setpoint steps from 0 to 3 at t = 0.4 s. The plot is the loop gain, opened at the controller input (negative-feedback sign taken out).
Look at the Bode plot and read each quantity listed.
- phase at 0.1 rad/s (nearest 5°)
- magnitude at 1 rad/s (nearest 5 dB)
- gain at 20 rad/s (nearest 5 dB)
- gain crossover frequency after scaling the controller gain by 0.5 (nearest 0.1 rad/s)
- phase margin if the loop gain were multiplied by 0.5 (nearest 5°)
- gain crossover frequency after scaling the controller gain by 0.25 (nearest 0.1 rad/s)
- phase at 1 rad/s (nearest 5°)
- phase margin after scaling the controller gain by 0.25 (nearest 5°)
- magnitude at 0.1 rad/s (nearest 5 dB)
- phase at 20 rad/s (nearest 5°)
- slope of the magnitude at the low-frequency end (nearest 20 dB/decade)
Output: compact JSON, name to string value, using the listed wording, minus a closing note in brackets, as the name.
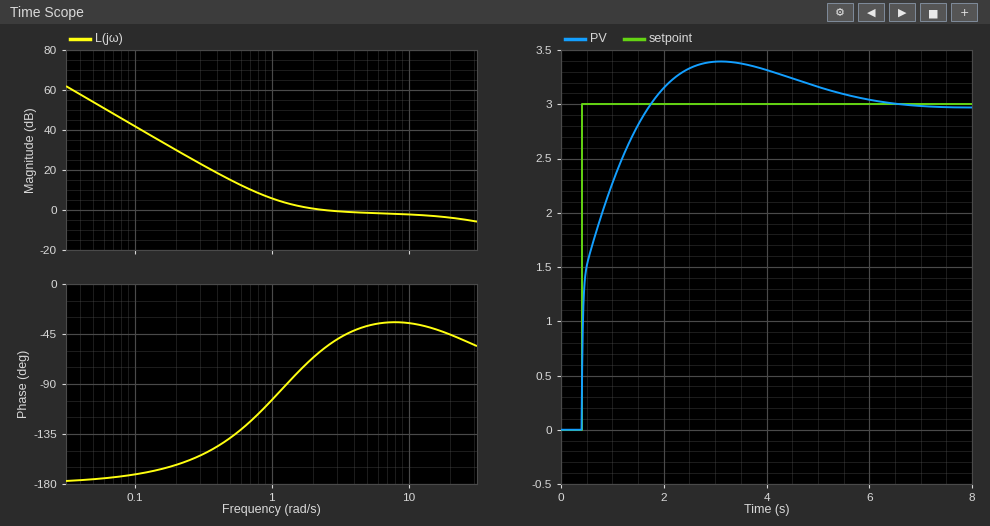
{"phase at 0.1 rad/s": "-170°", "magnitude at 1 rad/s": "5 dB", "gain at 20 rad/s": "-5 dB", "gain crossover frequency after scaling the controller gain by 0.5": "1.0 rad/s", "phase margin if the loop gain were multiplied by 0.5": "75°", "gain crossover frequency after scaling the controller gain by 0.25": "0.6 rad/s", "phase at 1 rad/s": "-105°", "phase margin after scaling the controller gain by 0.25": "50°", "magnitude at 0.1 rad/s": "40 dB", "phase at 20 rad/s": "-45°", "slope of the magnitude at the low-frequency end": "-40 dB/decade"}
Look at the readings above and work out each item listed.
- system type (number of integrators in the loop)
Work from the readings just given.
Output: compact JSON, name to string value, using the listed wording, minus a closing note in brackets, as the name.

{"system type": "2"}
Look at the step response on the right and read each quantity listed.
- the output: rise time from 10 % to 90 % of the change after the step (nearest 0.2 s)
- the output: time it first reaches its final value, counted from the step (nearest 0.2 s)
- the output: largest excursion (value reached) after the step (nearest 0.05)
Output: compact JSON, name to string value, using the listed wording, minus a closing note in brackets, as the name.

{"the output: rise time from 10 % to 90 % of the change after the step": "1.0 s", "the output: time it first reaches its final value, counted from the step": "1.4 s", "the output: largest excursion (value reached) after the step": "3.40"}
